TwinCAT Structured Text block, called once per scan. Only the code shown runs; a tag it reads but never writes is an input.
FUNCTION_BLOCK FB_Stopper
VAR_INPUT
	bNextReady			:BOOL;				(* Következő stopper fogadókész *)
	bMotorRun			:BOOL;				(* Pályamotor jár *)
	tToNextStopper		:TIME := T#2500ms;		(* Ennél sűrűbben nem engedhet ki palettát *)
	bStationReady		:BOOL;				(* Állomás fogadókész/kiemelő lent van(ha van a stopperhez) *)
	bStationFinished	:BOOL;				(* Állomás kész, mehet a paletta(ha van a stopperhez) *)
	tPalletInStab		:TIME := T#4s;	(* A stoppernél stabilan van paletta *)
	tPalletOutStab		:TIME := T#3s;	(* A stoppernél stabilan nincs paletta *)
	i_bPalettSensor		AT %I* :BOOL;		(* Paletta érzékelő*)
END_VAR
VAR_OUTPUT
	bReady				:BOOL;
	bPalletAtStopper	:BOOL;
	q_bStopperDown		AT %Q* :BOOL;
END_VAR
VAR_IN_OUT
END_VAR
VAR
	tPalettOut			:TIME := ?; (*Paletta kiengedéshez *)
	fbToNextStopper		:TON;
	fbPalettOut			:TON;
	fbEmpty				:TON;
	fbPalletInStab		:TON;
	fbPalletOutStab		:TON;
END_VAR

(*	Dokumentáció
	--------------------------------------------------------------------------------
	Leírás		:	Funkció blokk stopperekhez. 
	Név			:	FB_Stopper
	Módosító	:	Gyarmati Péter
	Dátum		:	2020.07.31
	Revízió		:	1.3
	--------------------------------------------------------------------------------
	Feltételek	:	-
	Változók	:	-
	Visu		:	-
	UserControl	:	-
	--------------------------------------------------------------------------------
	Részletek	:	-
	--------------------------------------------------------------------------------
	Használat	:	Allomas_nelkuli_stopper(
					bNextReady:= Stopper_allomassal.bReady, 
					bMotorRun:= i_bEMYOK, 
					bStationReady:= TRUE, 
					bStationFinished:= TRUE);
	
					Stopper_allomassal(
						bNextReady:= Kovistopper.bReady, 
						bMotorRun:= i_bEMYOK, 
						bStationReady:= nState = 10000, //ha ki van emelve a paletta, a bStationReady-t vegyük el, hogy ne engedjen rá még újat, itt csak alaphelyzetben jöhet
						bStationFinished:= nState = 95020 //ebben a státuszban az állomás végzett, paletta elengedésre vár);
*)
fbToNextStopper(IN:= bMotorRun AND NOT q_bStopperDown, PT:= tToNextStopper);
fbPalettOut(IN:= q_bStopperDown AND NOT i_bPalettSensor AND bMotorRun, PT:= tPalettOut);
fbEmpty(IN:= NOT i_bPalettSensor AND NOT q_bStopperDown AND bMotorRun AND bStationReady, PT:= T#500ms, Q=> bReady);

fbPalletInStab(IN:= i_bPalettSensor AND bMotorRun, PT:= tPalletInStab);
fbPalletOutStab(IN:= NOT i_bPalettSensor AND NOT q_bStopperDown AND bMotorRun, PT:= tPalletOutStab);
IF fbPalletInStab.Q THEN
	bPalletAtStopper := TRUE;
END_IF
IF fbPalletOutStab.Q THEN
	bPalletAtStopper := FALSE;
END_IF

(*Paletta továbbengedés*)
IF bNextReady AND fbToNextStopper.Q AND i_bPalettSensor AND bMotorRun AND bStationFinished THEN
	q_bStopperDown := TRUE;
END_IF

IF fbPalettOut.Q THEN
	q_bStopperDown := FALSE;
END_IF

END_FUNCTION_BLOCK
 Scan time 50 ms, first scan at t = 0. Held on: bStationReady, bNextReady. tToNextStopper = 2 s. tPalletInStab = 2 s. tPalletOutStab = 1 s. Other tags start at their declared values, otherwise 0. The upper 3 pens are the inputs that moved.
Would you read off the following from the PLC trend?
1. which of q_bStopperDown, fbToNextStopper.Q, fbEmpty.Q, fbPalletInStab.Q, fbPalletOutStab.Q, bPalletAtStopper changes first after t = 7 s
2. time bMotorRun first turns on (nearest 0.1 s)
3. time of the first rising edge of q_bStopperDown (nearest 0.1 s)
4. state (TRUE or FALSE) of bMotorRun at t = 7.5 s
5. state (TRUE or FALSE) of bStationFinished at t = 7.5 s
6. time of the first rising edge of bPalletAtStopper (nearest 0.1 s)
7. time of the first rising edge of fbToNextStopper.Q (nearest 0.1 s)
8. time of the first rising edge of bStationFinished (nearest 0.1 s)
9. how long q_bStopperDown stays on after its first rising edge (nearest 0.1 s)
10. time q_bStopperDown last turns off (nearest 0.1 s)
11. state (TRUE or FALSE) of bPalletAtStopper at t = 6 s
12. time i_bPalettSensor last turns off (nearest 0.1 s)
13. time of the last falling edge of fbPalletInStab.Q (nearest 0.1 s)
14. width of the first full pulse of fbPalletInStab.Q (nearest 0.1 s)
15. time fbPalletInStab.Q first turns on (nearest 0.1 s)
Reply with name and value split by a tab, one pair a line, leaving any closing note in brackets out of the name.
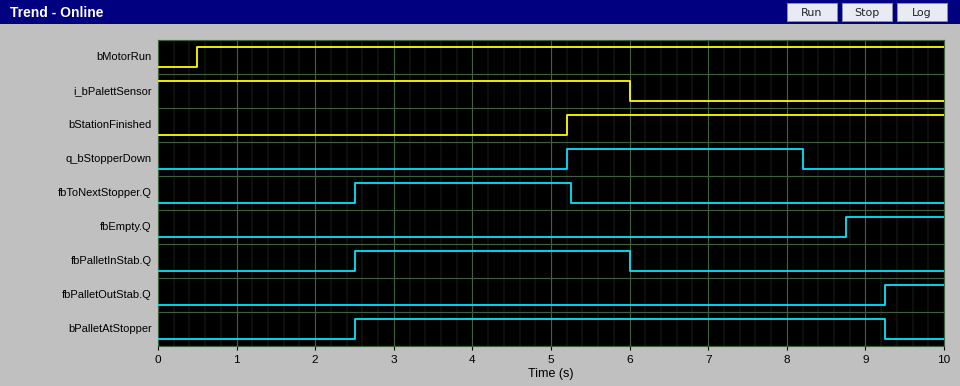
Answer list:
which of q_bStopperDown, fbToNextStopper.Q, fbEmpty.Q, fbPalletInStab.Q, fbPalletOutStab.Q, bPalletAtStopper changes first after t = 7 s	q_bStopperDown
time bMotorRun first turns on	0.5 s
time of the first rising edge of q_bStopperDown	5.2 s
state (TRUE or FALSE) of bMotorRun at t = 7.5 s	TRUE
state (TRUE or FALSE) of bStationFinished at t = 7.5 s	TRUE
time of the first rising edge of bPalletAtStopper	2.5 s
time of the first rising edge of fbToNextStopper.Q	2.5 s
time of the first rising edge of bStationFinished	5.2 s
how long q_bStopperDown stays on after its first rising edge	3.0 s
time q_bStopperDown last turns off	8.2 s
state (TRUE or FALSE) of bPalletAtStopper at t = 6 s	TRUE
time i_bPalettSensor last turns off	6.0 s
time of the last falling edge of fbPalletInStab.Q	6.0 s
width of the first full pulse of fbPalletInStab.Q	3.5 s
time fbPalletInStab.Q first turns on	2.5 s
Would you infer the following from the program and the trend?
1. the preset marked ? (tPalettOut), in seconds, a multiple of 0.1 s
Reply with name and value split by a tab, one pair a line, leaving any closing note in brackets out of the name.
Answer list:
the preset marked ? (tPalettOut), in seconds, a multiple of 0.1 s	2.2 s
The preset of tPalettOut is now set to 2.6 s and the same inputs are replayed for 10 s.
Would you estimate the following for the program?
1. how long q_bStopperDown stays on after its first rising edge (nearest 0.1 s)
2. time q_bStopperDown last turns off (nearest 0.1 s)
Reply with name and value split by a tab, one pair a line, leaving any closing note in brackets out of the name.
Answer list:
how long q_bStopperDown stays on after its first rising edge	3.4 s
time q_bStopperDown last turns off	8.6 s
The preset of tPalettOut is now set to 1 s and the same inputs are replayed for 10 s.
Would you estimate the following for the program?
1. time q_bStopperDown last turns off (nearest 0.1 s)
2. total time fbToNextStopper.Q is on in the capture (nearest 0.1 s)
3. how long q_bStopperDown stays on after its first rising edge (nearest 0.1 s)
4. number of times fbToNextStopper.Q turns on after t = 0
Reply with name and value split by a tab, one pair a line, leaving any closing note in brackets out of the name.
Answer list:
time q_bStopperDown last turns off	7.0 s
total time fbToNextStopper.Q is on in the capture	3.7 s
how long q_bStopperDown stays on after its first rising edge	1.8 s
number of times fbToNextStopper.Q turns on after t = 0	2
